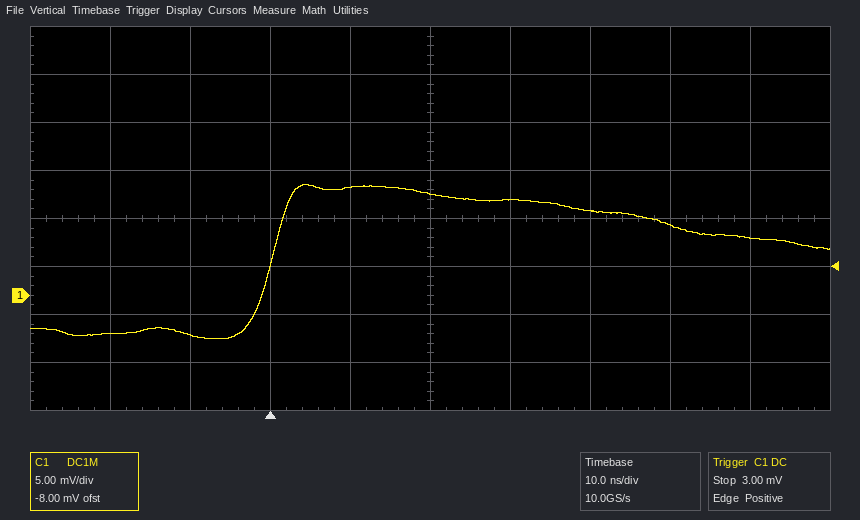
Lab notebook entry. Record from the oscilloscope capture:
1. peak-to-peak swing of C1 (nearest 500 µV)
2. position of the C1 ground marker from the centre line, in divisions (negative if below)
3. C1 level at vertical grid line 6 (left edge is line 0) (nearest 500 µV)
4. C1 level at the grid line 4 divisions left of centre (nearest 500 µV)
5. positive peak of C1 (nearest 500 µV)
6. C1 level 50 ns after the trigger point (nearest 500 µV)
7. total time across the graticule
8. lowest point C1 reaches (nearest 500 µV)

16.0 mV
-1.6 div
10.0 mV
-4.0 mV
11.5 mV
7.5 mV
100 ns
-4.5 mV
